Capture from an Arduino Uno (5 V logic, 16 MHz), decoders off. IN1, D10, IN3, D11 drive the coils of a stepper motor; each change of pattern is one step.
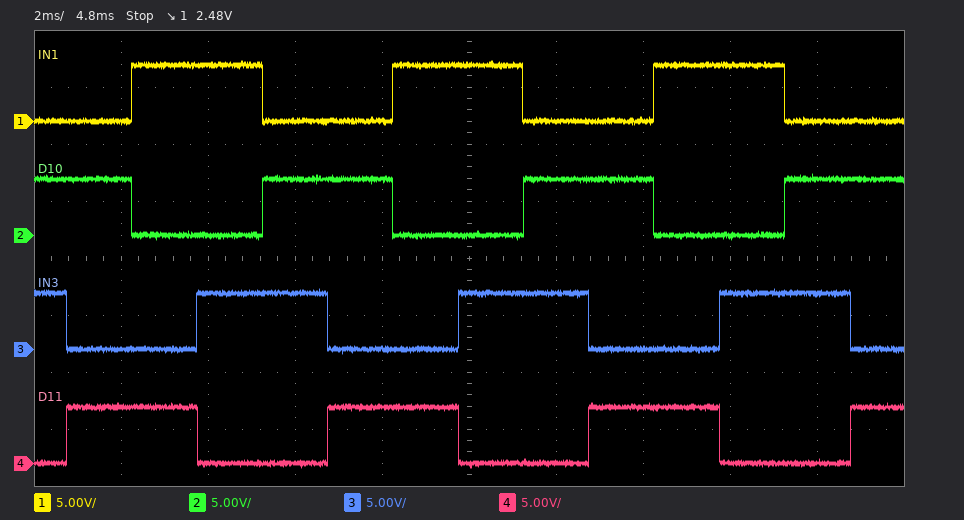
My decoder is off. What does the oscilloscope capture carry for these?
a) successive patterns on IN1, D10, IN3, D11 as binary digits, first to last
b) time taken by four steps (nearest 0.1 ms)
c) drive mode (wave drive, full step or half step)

0110 0101 1001 1010 0110 0101 1001 1010 0110 0101 1001 1010 0110 0101
6.0 ms
full step
